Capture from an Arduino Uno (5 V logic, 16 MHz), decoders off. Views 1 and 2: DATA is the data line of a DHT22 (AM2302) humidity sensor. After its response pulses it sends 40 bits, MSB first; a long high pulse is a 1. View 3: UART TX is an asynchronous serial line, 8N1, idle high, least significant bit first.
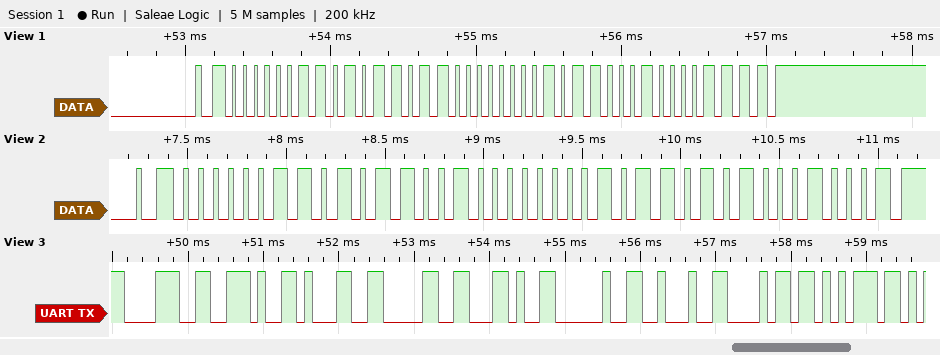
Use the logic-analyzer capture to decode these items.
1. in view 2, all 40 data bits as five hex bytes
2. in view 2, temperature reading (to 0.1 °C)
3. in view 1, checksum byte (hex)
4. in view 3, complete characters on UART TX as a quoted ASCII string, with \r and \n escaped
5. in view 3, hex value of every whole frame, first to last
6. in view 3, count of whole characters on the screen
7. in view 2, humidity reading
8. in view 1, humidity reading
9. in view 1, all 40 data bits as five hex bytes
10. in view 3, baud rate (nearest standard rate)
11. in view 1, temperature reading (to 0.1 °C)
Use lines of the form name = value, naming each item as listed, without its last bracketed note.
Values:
in view 2, all 40 data bits as five hex bytes = 03 59 00 B5 11
in view 2, temperature reading = 18.1 °C
in view 1, checksum byte = 0x0F
in view 3, complete characters on UART TX as a quoted ASCII string, with \r and \n escaped = "8.10, \"hu"
in view 3, hex value of every whole frame, first to last = 38 2E 31 30 2C 20 22 68 75
in view 3, count of whole characters on the screen = 9
in view 2, humidity reading = 85.7 %
in view 1, humidity reading = 85.9 %
in view 1, all 40 data bits as five hex bytes = 03 5B 00 B1 0F
in view 3, baud rate = 9600 baud
in view 1, temperature reading = 17.7 °C
